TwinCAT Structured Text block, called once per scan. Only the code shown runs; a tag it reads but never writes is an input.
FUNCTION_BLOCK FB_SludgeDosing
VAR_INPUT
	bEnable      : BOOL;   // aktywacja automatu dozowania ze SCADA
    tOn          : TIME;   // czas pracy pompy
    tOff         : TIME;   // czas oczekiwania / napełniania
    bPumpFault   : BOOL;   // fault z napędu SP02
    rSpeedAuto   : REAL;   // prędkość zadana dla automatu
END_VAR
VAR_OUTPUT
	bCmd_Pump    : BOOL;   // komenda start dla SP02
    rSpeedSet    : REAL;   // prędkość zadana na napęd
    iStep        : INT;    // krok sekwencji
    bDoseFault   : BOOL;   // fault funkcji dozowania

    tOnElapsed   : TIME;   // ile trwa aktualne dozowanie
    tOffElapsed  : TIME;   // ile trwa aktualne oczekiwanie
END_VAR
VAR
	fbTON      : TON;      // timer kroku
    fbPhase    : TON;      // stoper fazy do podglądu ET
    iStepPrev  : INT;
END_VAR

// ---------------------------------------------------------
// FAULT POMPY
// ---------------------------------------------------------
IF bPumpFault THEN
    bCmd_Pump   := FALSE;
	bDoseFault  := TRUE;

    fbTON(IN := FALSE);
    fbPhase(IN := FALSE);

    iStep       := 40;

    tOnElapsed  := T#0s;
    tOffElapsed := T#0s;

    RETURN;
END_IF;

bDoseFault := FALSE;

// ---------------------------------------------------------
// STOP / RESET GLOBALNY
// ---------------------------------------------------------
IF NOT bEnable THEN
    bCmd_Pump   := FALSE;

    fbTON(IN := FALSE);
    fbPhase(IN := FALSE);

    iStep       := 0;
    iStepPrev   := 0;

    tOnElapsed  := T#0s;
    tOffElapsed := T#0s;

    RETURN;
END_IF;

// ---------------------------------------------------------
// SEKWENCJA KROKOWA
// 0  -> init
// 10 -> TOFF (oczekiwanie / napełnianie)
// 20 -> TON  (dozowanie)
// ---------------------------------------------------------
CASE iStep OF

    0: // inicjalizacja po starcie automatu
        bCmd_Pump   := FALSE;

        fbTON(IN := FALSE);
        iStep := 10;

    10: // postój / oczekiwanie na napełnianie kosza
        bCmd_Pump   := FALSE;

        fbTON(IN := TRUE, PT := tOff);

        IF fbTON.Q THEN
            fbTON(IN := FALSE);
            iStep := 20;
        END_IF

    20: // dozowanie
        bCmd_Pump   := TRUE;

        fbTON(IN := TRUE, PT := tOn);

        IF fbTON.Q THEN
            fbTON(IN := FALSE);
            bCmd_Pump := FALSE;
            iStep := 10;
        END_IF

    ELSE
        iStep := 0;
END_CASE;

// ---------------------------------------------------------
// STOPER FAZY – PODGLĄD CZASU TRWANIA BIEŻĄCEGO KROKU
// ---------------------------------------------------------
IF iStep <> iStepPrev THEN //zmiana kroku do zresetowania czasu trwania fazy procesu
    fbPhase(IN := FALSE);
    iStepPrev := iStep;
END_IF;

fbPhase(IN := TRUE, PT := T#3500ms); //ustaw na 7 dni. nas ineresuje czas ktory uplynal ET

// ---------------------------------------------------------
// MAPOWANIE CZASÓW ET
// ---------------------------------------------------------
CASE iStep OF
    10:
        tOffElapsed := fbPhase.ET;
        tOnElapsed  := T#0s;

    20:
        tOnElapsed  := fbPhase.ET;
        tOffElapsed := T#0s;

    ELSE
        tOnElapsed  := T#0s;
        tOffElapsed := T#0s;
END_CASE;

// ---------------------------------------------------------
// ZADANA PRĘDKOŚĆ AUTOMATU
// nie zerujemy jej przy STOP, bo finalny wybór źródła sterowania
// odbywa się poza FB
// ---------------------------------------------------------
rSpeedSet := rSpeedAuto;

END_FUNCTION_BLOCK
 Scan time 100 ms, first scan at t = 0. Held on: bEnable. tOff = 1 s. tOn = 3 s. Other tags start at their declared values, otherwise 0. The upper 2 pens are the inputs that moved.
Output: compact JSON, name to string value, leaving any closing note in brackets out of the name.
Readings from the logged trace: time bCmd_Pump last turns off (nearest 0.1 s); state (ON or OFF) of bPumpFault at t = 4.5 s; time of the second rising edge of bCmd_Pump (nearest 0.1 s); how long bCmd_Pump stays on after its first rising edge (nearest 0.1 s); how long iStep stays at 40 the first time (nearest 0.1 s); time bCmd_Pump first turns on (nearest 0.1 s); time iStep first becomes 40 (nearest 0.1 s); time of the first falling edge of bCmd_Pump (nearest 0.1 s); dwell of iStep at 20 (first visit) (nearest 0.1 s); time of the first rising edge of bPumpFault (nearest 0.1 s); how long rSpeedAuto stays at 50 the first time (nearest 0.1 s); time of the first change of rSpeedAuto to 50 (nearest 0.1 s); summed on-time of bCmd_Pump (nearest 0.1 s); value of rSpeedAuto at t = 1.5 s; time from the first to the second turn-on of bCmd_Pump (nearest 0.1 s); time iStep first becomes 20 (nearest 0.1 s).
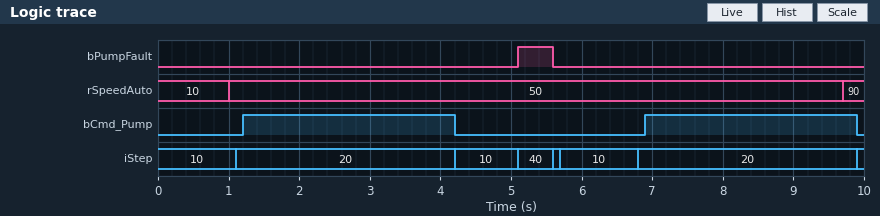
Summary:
{"time bCmd_Pump last turns off": "9.9 s", "state (ON or OFF) of bPumpFault at t = 4.5 s": "OFF", "time of the second rising edge of bCmd_Pump": "6.9 s", "how long bCmd_Pump stays on after its first rising edge": "3.0 s", "how long iStep stays at 40 the first time": "0.5 s", "time bCmd_Pump first turns on": "1.2 s", "time iStep first becomes 40": "5.1 s", "time of the first falling edge of bCmd_Pump": "4.2 s", "dwell of iStep at 20 (first visit)": "3.1 s", "time of the first rising edge of bPumpFault": "5.1 s", "how long rSpeedAuto stays at 50 the first time": "8.7 s", "time of the first change of rSpeedAuto to 50": "1.0 s", "summed on-time of bCmd_Pump": "6.0 s", "value of rSpeedAuto at t = 1.5 s": "50", "time from the first to the second turn-on of bCmd_Pump": "5.7 s", "time iStep first becomes 20": "1.1 s"}
